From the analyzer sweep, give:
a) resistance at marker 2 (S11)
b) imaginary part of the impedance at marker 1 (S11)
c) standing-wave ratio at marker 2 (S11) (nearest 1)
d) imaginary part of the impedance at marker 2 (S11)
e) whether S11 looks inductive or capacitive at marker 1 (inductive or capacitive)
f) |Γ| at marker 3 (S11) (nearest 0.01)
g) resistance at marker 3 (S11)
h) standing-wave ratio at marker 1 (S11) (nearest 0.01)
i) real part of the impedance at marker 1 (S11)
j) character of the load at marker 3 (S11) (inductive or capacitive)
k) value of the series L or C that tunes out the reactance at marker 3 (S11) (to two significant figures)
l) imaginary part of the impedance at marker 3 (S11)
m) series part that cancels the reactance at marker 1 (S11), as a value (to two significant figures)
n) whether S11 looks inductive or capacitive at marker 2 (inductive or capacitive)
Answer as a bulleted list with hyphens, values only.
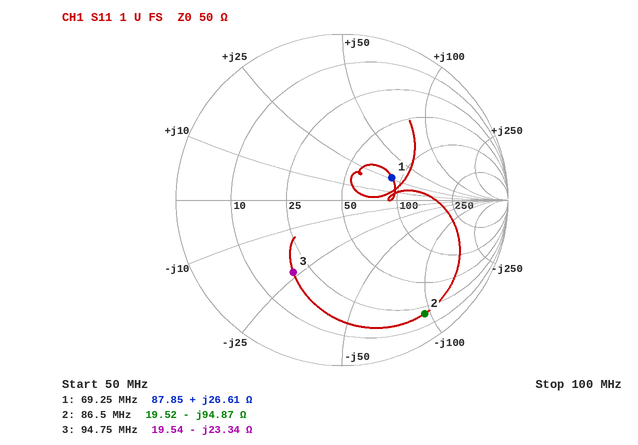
- 19.52 Ω
- +26.61 Ω
- 12
- -94.87 Ω
- inductive
- 0.52
- 19.54 Ω
- 1.98
- 87.85 Ω
- capacitive
- 39 nH
- -23.34 Ω
- 86 pF
- capacitive
